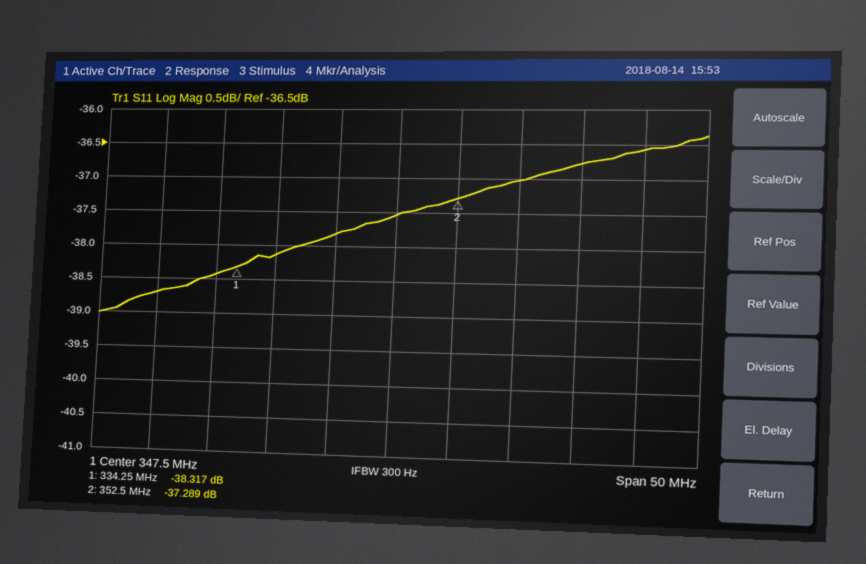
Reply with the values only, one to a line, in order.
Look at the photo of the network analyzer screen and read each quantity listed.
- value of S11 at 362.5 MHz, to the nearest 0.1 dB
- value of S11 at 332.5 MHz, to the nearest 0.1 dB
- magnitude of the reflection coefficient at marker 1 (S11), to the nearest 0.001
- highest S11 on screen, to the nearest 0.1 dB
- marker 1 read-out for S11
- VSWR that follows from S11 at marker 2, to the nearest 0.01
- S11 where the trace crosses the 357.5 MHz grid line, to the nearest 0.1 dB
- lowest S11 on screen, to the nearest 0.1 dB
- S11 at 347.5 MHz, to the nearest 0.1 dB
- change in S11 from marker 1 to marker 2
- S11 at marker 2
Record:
-36.8 dB
-38.4 dB
0.012
-36.4 dB
-38.317 dB
1.03
-37.0 dB
-39.0 dB
-37.5 dB
1.028 dB
-37.289 dB
